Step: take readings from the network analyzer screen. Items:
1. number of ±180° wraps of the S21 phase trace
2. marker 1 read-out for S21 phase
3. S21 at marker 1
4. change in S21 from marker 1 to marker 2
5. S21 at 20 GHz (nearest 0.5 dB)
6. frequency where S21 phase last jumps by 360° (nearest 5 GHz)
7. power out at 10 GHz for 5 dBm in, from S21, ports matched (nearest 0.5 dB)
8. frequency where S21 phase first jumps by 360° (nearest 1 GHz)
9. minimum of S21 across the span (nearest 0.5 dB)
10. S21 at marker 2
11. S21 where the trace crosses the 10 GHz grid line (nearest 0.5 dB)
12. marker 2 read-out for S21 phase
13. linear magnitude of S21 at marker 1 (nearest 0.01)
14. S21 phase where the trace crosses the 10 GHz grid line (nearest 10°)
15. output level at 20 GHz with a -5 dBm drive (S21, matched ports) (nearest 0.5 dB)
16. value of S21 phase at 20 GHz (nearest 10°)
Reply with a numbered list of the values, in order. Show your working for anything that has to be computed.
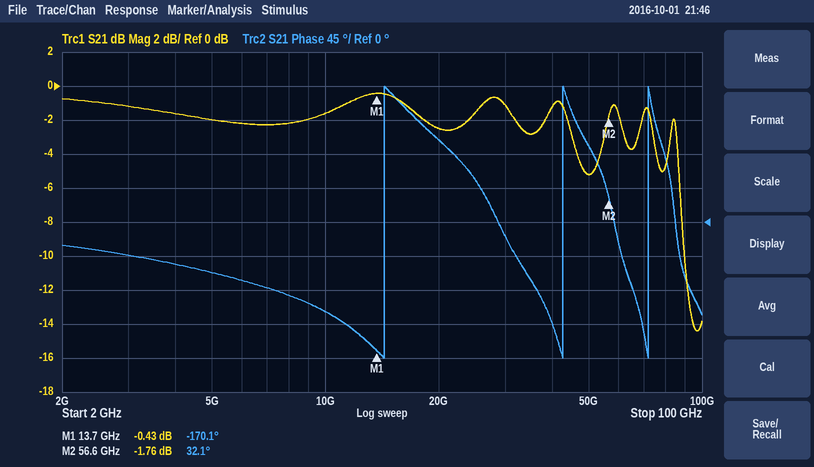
1. 3
2. -170.1°
3. -0.43 dB
4. -1.76 − (-0.43) = -1.33 dB
5. -2.5 dB
6. 70 GHz
7. 5 dBm + (-1.5 dB) = 3.5 dBm
8. 14 GHz
9. -14.5 dB
10. -1.76 dB
11. -1.5 dB
12. 32.1°
13. 10^(-0.43/20) ≈ 0.95
14. -120°
15. -5 dBm + (-2.5 dB) = -7.5 dBm
16. 110°
